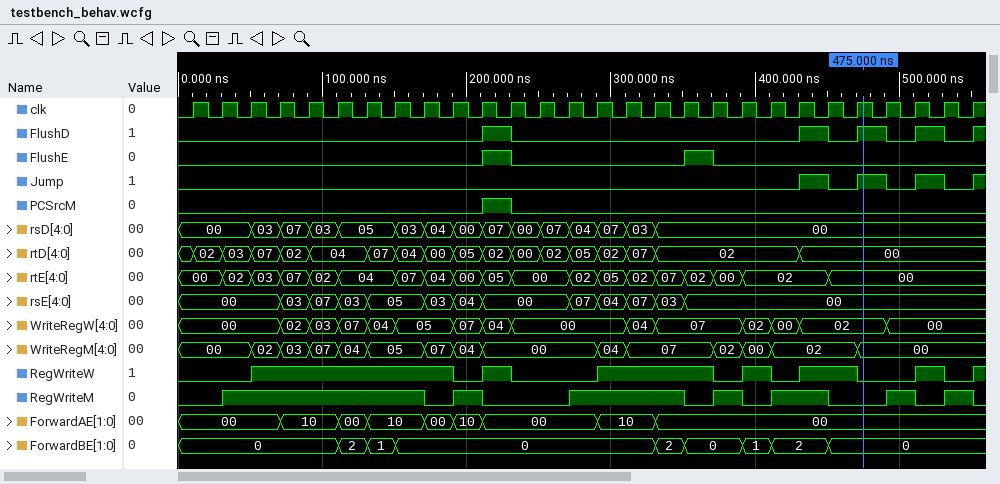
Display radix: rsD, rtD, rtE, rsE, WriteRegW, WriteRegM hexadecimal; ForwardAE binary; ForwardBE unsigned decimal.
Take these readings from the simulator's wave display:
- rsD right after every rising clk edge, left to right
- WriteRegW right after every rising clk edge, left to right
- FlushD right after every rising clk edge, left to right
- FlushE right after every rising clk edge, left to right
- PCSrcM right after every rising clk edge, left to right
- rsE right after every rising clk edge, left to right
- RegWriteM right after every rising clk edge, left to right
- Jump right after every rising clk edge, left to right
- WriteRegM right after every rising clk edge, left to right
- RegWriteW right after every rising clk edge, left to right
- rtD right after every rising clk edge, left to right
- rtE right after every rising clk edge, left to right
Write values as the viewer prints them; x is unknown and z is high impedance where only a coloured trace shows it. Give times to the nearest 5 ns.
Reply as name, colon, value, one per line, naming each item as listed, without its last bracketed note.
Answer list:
rsD right after every rising clk edge, left to right: 00, 00, 03, 07, 03, 05, 05, 03, 04, 00, 07, 00, 07, 04, 07, 03, 00, 00, 00, 00, 00, 00, 00, 00, 00, 00, 00, 00
WriteRegW right after every rising clk edge, left to right: 00, 00, 00, 02, 03, 07, 04, 05, 05, 07, 04, 00, 00, 00, 00, 04, 07, 07, 07, 02, 00, 02, 02, 02, 00, 00, 00, 00
FlushD right after every rising clk edge, left to right: 0 0 0 0 0 0 0 0 0 0 1 0 0 0 0 0 0 0 0 0 0 1 0 1 0 1 0 1
FlushE right after every rising clk edge, left to right: 0 0 0 0 0 0 0 0 0 0 1 0 0 0 0 0 0 1 0 0 0 0 0 0 0 0 0 0
PCSrcM right after every rising clk edge, left to right: 0 0 0 0 0 0 0 0 0 0 1 0 0 0 0 0 0 0 0 0 0 0 0 0 0 0 0 0
rsE right after every rising clk edge, left to right: 00, 00, 00, 03, 07, 03, 05, 05, 03, 04, 00, 00, 00, 07, 04, 07, 03, 00, 00, 00, 00, 00, 00, 00, 00, 00, 00, 00
RegWriteM right after every rising clk edge, left to right: 0 1 1 1 1 1 1 1 0 1 0 0 0 1 1 1 1 0 1 0 1 1 0 0 1 0 1 0
Jump right after every rising clk edge, left to right: 0 0 0 0 0 0 0 0 0 0 0 0 0 0 0 0 0 0 0 0 0 1 0 1 0 1 0 1
WriteRegM right after every rising clk edge, left to right: 00, 00, 02, 03, 07, 04, 05, 05, 07, 04, 00, 00, 00, 00, 04, 07, 07, 07, 02, 00, 02, 02, 02, 00, 00, 00, 00, 00
RegWriteW right after every rising clk edge, left to right: 0 0 1 1 1 1 1 1 1 0 1 0 0 0 1 1 1 1 0 1 0 1 1 0 0 1 0 1
rtD right after every rising clk edge, left to right: 02, 03, 07, 02, 04, 04, 07, 04, 00, 05, 02, 00, 02, 05, 02, 07, 02, 02, 02, 02, 02, 00, 00, 00, 00, 00, 00, 00
rtE right after every rising clk edge, left to right: 00, 02, 03, 07, 02, 04, 04, 07, 04, 00, 05, 00, 00, 02, 05, 02, 07, 02, 00, 02, 02, 02, 00, 00, 00, 00, 00, 00
